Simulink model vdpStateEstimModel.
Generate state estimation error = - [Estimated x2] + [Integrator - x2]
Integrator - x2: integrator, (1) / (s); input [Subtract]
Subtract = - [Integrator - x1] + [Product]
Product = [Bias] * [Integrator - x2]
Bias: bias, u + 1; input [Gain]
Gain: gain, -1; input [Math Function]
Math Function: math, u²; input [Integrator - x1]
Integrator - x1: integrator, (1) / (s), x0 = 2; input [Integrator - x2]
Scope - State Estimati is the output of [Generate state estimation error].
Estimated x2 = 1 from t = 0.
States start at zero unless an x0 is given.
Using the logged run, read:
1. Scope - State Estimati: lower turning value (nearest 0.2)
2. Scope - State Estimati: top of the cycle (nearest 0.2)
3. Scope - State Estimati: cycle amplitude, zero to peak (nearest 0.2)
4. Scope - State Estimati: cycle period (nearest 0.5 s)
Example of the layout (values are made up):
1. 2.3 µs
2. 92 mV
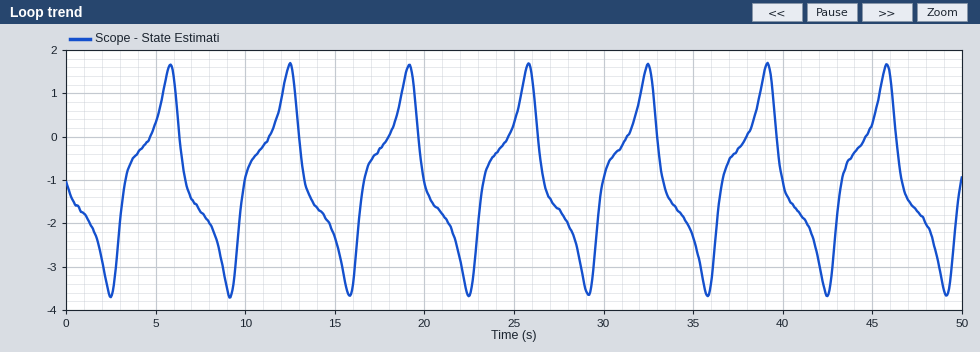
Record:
1. -3.6
2. 1.6
3. 2.6
4. 6.5 s
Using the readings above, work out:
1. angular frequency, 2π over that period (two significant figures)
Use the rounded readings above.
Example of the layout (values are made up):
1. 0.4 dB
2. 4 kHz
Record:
1. 0.97 rad/s
